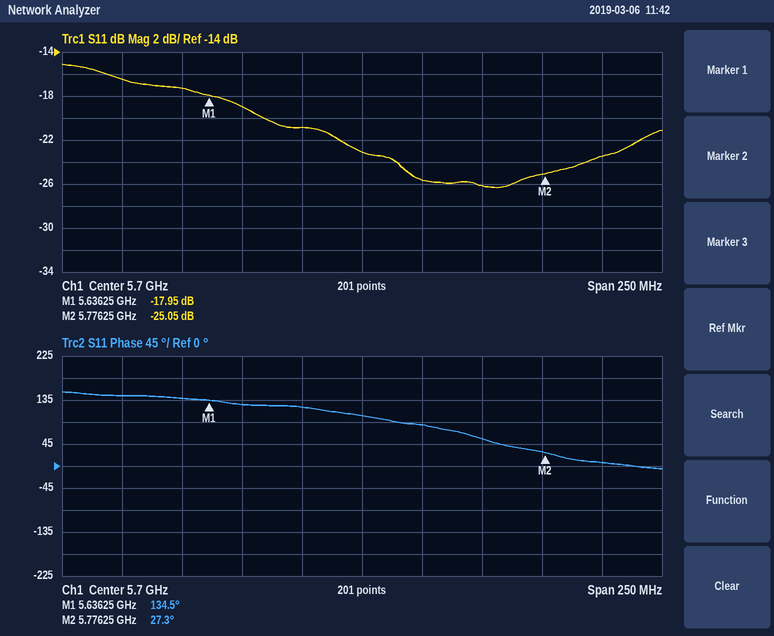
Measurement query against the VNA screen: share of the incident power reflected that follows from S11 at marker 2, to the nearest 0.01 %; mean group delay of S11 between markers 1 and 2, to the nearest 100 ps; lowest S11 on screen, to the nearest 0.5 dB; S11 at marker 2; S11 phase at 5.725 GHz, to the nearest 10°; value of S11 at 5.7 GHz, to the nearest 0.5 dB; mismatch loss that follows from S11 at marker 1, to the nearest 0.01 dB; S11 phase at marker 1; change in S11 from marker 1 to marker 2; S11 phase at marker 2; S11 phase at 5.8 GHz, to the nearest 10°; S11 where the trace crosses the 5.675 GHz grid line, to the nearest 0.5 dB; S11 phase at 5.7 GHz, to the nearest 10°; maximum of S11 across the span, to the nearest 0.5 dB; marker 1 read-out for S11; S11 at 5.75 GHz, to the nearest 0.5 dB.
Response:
0.31 %
2.1 ns
-26.5 dB
-25.05 dB
80°
-23.0 dB
0.07 dB
134.5°
-7.10 dB
27.3°
10°
-21.0 dB
100°
-15.0 dB
-17.95 dB
-26.0 dB
